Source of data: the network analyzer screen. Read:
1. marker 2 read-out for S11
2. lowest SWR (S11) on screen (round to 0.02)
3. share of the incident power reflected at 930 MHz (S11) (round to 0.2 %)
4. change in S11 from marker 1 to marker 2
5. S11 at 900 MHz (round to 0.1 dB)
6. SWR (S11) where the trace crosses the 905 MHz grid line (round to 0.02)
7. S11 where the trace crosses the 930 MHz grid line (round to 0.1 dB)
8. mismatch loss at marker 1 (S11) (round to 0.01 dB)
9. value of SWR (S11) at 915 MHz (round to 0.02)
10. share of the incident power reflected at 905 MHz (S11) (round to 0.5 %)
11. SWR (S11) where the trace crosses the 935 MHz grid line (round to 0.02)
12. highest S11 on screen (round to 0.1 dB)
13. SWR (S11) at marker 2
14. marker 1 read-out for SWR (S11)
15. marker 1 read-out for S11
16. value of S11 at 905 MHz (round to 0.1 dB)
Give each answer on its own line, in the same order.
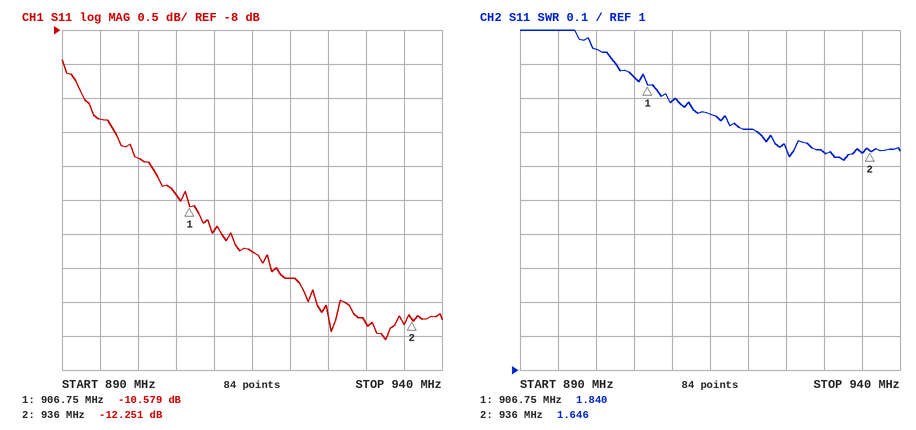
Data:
-12.251 dB
1.62
5.8 %
-1.672 dB
-9.9 dB
1.86
-12.3 dB
0.40 dB
1.76
9.0 %
1.64
-8.4 dB
1.646
1.840
-10.579 dB
-10.4 dB
